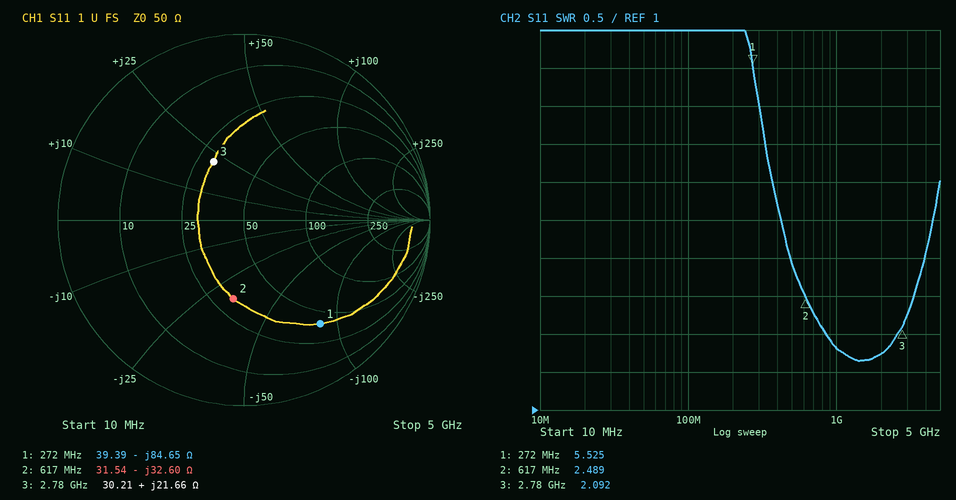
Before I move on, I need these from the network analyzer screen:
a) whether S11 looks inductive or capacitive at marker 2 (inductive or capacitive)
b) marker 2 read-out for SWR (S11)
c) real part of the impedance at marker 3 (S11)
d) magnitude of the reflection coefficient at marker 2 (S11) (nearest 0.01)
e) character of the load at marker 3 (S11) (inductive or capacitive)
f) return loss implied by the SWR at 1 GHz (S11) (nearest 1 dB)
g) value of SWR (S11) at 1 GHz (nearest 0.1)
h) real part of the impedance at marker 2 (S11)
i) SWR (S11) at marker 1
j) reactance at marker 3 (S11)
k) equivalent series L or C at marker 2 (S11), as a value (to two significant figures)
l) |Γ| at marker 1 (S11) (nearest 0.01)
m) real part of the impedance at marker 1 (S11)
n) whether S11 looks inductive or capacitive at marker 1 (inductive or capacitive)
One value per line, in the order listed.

capacitive
2.489
30.21 Ω
0.43
inductive
11 dB
1.8
31.54 Ω
5.525
+21.66 Ω
7.9 pF
0.69
39.39 Ω
capacitive
